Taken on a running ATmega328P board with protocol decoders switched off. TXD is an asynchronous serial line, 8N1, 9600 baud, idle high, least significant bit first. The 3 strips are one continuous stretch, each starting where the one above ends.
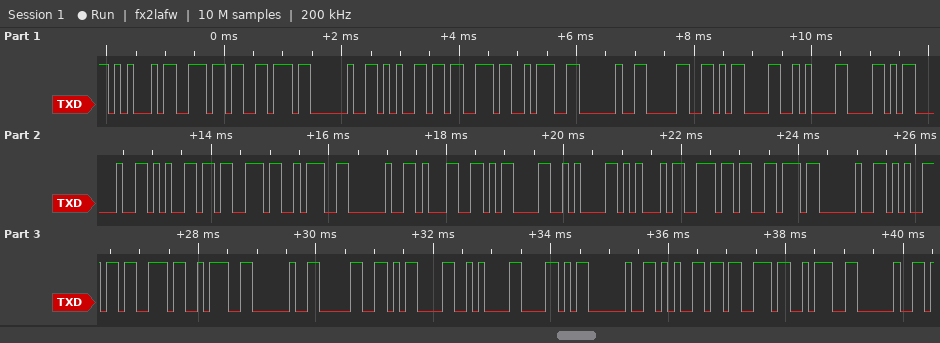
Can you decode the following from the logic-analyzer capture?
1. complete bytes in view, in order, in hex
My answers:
45 6E 76 20 65 73 3A 20 30 0D 0A 58 20 65 73 3A 20 31 0D 0A 45 6E 76 20 65 73 3A 20 30 0D 0A 58 20 65 73 3A 20
